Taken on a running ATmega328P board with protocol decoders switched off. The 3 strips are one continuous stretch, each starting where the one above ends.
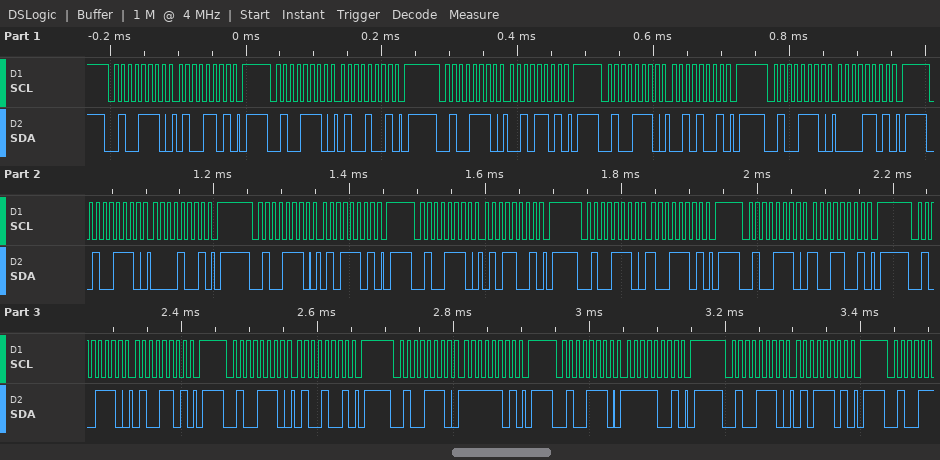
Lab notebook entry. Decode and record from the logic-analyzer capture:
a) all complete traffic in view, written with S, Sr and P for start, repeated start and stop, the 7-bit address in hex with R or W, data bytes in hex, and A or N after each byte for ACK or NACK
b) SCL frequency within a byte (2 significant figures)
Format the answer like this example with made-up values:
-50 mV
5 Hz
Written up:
S 27W A 4D A P S 27W A 49 A P S 27W A 2D A P S 27W A 29 A P S 27W A 0D A P S 27W A 09 A P S 27W A 5D A P S 27W A 59 A P S 27W A 9D A P S 27W A 99 A P S 27W A 4D A P S 27W A 49 A P S 27W A FD A P S 27W A F9 A P S 27W A 5D A P
100 kHz
